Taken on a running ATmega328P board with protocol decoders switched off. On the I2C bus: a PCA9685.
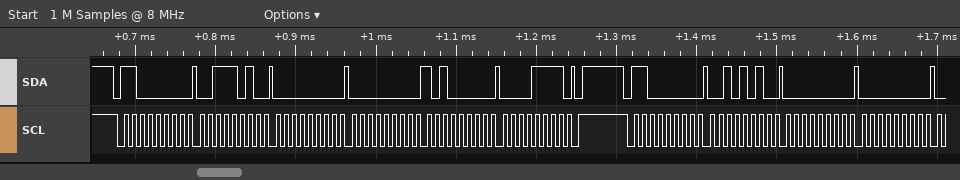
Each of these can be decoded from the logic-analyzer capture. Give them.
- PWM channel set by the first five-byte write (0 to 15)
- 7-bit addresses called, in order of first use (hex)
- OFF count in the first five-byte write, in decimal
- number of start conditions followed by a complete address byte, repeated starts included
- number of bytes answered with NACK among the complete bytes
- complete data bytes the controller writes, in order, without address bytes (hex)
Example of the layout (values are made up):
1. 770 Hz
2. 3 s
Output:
1. 13
2. 0x60
3. 4000
4. 2
5. 0
6. 3A 00 00 A0 0F 2A 00 00
